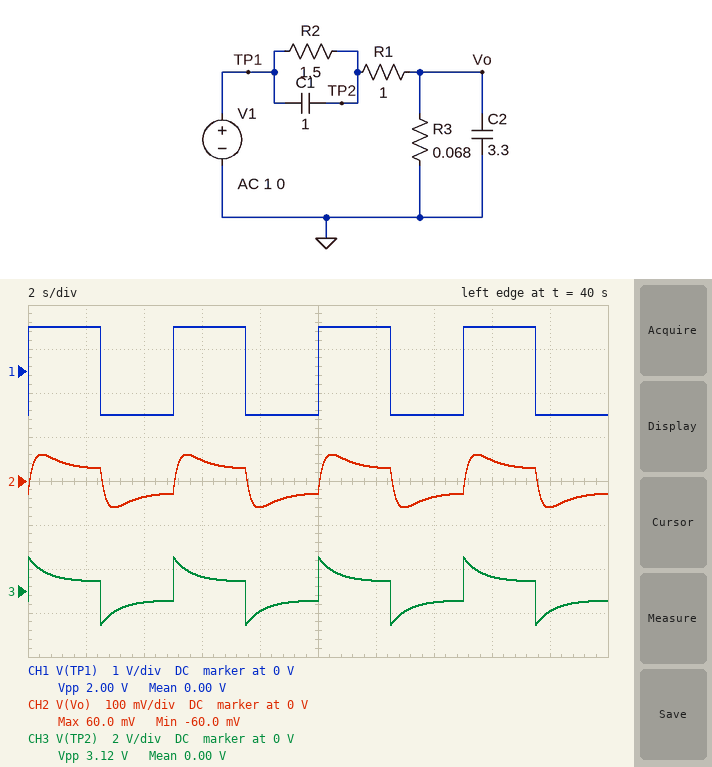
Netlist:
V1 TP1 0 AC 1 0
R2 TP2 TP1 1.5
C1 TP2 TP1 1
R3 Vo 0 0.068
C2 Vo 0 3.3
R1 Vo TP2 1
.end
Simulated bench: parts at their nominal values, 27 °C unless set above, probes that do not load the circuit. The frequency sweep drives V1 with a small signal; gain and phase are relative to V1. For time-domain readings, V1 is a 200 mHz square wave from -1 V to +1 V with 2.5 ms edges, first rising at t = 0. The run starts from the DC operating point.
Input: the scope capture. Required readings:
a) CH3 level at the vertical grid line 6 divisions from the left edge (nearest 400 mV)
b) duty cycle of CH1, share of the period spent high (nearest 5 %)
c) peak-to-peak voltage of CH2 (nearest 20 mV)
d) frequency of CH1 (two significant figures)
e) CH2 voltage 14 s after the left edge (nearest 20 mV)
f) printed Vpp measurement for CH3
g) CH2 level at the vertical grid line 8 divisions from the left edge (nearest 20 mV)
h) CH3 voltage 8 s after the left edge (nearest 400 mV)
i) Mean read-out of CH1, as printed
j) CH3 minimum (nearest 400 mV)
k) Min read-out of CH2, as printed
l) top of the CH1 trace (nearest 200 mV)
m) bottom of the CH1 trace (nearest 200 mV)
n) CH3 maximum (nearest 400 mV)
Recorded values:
400 mV
50 %
120 mV
200 mHz
-40 mV
3.12 V
40 mV
-800 mV
0.00 V
-1.6 V
-60.0 mV
1.0 V
-1.0 V
1.6 V
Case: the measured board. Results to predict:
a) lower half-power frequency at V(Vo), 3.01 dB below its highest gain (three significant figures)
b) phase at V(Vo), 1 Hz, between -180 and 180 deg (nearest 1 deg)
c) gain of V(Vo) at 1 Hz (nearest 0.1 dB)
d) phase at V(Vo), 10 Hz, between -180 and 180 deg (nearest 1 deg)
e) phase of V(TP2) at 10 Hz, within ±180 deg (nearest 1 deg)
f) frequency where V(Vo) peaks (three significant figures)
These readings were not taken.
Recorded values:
108 mHz
-44 deg
-28.6 dB
-85 deg
1 deg
403 mHz
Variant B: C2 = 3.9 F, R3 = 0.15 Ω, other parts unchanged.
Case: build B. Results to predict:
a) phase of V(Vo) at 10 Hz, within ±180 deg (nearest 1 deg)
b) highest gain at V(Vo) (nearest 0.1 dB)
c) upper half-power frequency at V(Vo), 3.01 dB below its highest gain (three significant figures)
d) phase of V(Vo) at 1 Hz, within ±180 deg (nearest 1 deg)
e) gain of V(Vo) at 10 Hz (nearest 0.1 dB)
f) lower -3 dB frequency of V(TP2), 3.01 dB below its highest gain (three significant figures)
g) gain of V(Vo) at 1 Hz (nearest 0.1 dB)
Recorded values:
-87 deg
-22.3 dB
623 mHz
-64 deg
-47.8 dB
211 mHz
-28.5 dB
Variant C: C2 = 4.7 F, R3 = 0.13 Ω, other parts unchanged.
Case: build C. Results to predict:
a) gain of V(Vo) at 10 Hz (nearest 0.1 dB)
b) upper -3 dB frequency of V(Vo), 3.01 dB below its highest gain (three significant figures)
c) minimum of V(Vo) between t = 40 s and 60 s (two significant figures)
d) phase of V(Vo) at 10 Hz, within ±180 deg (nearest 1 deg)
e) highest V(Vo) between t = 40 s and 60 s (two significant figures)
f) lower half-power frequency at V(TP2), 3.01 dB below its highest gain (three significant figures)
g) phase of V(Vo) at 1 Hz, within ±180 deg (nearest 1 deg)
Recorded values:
-49.4 dB
602 mHz
-73 mV
-87 deg
73 mV
213 mHz
-65 deg
